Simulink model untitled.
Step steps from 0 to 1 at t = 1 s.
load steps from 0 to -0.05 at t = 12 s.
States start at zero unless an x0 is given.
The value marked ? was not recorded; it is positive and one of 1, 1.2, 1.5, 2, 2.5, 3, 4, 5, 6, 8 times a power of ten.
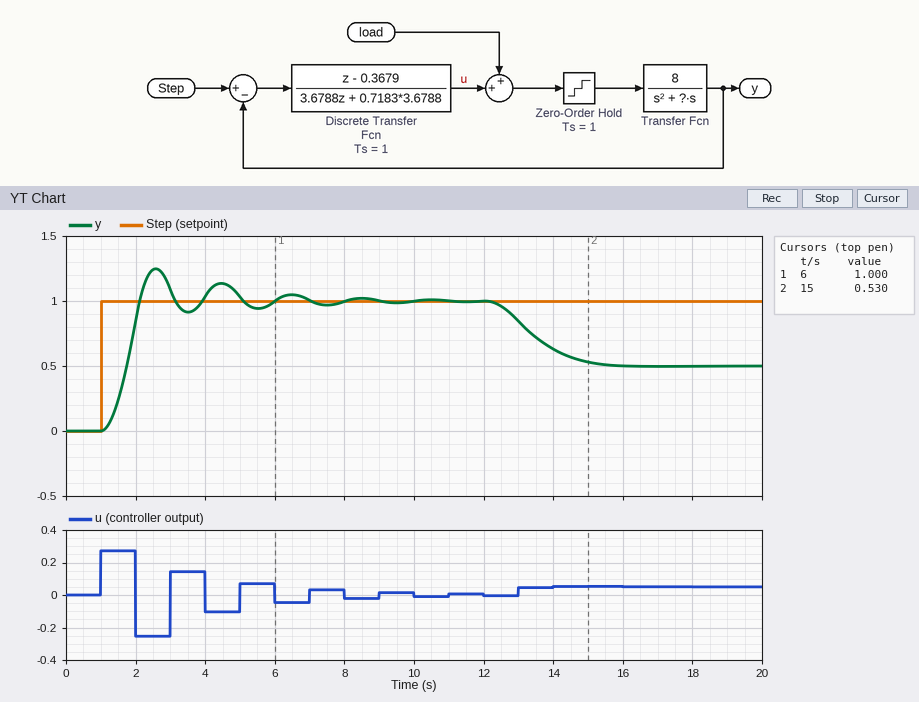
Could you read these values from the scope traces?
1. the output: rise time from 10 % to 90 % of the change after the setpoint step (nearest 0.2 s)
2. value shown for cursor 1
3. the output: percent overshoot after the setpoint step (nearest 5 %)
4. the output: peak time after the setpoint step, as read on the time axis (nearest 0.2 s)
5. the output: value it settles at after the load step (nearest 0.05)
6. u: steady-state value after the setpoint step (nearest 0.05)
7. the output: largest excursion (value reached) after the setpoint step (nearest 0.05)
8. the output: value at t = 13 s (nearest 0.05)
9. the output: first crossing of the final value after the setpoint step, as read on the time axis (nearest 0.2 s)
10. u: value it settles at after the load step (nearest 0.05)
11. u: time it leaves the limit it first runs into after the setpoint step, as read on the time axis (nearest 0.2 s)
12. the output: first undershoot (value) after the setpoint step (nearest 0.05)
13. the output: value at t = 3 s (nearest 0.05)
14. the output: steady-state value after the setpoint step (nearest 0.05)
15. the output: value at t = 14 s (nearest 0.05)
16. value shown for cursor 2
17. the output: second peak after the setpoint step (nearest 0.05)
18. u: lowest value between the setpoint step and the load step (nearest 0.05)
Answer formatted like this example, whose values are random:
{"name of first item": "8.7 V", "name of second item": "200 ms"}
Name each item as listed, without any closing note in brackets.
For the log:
{"the output: rise time from 10 % to 90 % of the change after the setpoint step": "0.8 s", "value shown for cursor 1": "1.000", "the output: percent overshoot after the setpoint step": "25 %", "the output: peak time after the setpoint step, as read on the time axis": "2.6 s", "the output: value it settles at after the load step": "0.50", "u: steady-state value after the setpoint step": "0.00", "the output: largest excursion (value reached) after the setpoint step": "1.25", "the output: value at t = 13 s": "0.85", "the output: first crossing of the final value after the setpoint step, as read on the time axis": "2.2 s", "u: value it settles at after the load step": "0.05", "u: time it leaves the limit it first runs into after the setpoint step, as read on the time axis": "2.0 s", "the output: first undershoot (value) after the setpoint step": "0.90", "the output: value at t = 3 s": "1.10", "the output: steady-state value after the setpoint step": "1.00", "the output: value at t = 14 s": "0.65", "value shown for cursor 2": "0.530", "the output: second peak after the setpoint step": "1.15", "u: lowest value between the setpoint step and the load step": "-0.25"}
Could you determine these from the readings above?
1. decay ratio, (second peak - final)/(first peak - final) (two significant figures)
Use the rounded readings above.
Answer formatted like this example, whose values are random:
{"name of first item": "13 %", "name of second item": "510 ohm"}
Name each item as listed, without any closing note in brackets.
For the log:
{"decay ratio, (second peak - final)/(first peak - final)": "0.60"}
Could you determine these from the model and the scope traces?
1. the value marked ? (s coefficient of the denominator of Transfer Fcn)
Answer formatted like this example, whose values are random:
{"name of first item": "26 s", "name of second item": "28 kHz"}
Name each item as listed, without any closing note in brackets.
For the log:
{"the value marked ?": "0.8"}
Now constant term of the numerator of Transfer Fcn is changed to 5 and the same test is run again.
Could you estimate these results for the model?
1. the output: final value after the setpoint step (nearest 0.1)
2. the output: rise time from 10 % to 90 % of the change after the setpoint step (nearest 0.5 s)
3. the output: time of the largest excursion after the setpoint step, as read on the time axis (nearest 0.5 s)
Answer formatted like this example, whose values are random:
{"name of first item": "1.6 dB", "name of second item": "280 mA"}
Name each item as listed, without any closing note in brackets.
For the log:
{"the output: final value after the setpoint step": "1.0", "the output: rise time from 10 % to 90 % of the change after the setpoint step": "2.5 s", "the output: time of the largest excursion after the setpoint step, as read on the time axis": "4.5 s"}
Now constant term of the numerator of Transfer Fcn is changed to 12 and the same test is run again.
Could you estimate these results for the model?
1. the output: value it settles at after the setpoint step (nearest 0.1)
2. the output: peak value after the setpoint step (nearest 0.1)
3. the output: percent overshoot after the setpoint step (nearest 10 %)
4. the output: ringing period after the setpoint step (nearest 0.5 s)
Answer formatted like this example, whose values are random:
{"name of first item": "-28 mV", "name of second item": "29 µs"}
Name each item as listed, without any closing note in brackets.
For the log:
{"the output: value it settles at after the setpoint step": "1.0", "the output: peak value after the setpoint step": "1.7", "the output: percent overshoot after the setpoint step": "70 %", "the output: ringing period after the setpoint step": "2.0 s"}
